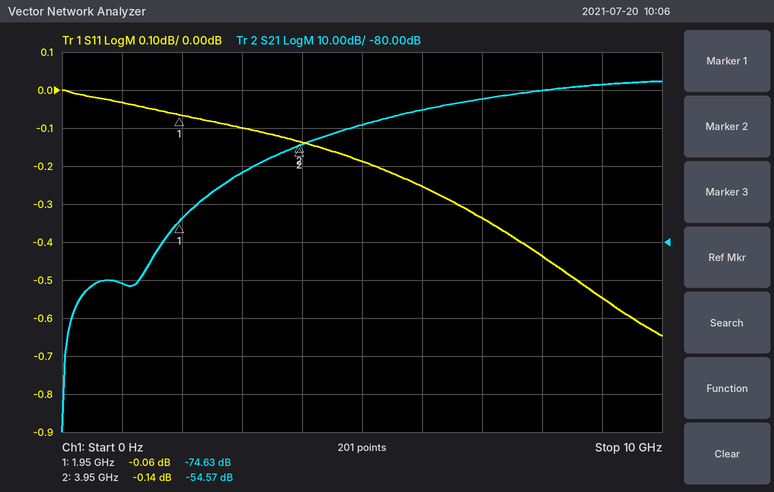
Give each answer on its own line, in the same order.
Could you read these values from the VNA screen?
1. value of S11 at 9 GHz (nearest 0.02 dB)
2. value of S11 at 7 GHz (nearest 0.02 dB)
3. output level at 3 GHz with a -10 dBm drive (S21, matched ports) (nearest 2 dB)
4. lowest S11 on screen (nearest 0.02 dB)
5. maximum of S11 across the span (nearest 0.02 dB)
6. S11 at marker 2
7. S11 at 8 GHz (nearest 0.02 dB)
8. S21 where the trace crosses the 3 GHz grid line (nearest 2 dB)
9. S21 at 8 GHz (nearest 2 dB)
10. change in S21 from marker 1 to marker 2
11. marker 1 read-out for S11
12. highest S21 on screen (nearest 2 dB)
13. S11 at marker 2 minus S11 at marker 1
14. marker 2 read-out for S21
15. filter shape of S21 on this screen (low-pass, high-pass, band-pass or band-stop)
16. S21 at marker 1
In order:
-0.54 dB
-0.34 dB
-72 dBm
-0.64 dB
0.00 dB
-0.14 dB
-0.44 dB
-62 dB
-40 dB
20.06 dB
-0.06 dB
-38 dB
-0.08 dB
-54.57 dB
high-pass
-74.63 dB
